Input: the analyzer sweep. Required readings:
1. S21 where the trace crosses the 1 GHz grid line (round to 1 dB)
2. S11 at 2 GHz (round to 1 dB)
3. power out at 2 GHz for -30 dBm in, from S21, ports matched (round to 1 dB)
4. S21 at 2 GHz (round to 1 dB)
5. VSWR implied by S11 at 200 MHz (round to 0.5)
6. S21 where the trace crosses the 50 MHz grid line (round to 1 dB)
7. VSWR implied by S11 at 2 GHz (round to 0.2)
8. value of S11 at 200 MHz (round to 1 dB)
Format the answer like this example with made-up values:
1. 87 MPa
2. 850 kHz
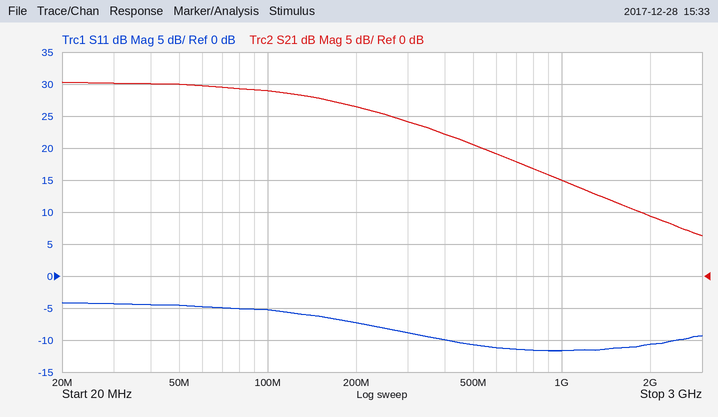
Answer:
1. 15 dB
2. -11 dB
3. -21 dBm
4. 9 dB
5. 2.5
6. 30 dB
7. 1.8
8. -7 dB
